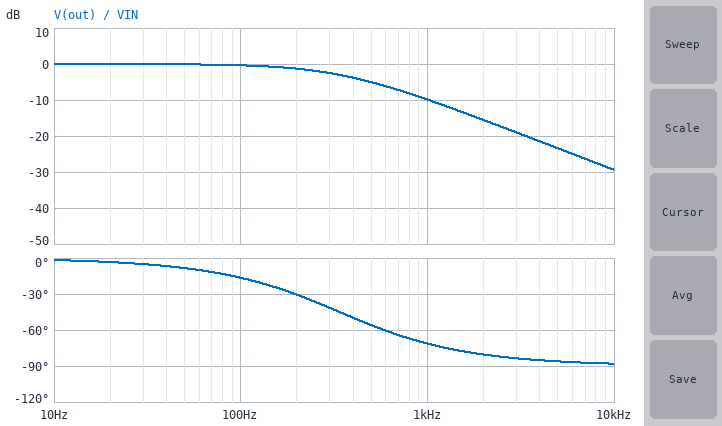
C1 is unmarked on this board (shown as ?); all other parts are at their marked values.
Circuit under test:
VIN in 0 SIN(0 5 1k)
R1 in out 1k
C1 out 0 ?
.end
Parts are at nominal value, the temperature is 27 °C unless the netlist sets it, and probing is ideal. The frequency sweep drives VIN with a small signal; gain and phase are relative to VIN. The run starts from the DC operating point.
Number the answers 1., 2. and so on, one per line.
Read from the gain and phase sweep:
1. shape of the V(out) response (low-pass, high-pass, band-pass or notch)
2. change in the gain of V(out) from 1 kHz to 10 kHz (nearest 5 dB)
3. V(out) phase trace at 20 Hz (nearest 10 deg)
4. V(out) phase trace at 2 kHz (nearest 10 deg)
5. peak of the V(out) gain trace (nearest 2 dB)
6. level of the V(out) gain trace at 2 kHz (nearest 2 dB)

1. low-pass
2. -20 dB
3. 0 deg
4. -80 deg
5. 0 dB
6. -16 dB
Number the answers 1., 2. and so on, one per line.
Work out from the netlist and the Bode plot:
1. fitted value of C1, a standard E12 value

1. 470 nF
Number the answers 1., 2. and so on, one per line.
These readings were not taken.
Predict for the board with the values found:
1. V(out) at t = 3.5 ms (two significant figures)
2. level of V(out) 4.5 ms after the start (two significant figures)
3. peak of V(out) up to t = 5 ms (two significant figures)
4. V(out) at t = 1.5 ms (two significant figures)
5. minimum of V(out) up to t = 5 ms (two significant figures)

1. 1.5 V
2. 1.5 V
3. 2.2 V
4. 1.6 V
5. -1.6 V
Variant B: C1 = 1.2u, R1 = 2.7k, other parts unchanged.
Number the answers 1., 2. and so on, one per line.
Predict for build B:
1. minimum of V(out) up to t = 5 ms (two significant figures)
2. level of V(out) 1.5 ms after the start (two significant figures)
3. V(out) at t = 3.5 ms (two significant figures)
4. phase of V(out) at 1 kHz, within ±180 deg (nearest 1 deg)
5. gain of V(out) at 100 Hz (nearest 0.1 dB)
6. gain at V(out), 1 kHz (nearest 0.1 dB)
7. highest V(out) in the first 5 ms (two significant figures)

1. -190 mV
2. 400 mV
3. 330 mV
4. -87 deg
5. -7.1 dB
6. -26.2 dB
7. 460 mV
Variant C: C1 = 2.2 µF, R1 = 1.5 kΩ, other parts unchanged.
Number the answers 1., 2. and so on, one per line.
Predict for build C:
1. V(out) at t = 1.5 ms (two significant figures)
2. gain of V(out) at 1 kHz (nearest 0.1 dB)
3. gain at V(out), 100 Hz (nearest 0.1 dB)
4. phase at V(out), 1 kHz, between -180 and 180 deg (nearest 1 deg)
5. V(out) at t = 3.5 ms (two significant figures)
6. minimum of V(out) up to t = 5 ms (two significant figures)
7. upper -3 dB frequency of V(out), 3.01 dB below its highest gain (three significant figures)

1. 390 mV
2. -26.3 dB
3. -7.2 dB
4. -87 deg
5. 320 mV
6. -190 mV
7. 48.2 Hz
